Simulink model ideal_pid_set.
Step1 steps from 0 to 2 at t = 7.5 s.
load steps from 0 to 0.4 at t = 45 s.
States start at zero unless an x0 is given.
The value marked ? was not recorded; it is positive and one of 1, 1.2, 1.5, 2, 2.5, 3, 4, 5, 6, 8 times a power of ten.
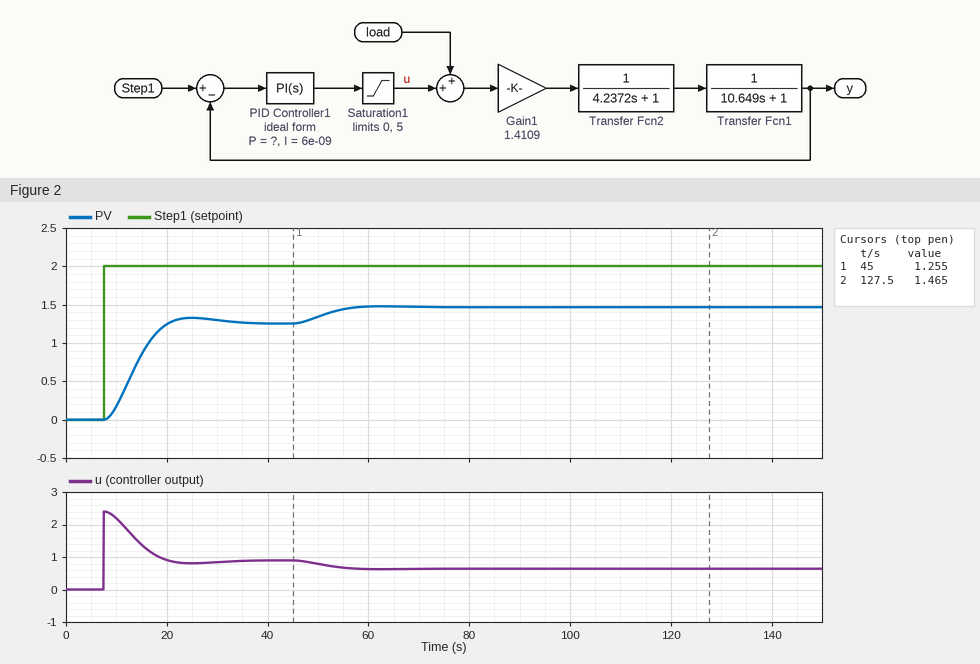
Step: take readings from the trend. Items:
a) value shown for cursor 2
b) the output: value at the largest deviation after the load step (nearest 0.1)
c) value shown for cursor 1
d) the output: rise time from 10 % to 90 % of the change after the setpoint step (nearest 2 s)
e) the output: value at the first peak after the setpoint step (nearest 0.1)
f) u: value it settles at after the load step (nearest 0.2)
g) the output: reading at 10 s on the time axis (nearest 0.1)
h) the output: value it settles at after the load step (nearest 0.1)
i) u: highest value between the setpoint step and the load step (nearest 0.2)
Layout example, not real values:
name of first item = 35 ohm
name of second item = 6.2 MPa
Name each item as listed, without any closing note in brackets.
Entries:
value shown for cursor 2 = 1.465
the output: value at the largest deviation after the load step = 1.5
value shown for cursor 1 = 1.255
the output: rise time from 10 % to 90 % of the change after the setpoint step = 8 s
the output: value at the first peak after the setpoint step = 1.3
u: value it settles at after the load step = 0.6
the output: reading at 10 s on the time axis = 0.2
the output: value it settles at after the load step = 1.5
u: highest value between the setpoint step and the load step = 2.4
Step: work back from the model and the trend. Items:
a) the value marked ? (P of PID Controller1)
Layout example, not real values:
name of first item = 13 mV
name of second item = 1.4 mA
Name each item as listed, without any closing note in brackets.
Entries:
the value marked ? = 1.2
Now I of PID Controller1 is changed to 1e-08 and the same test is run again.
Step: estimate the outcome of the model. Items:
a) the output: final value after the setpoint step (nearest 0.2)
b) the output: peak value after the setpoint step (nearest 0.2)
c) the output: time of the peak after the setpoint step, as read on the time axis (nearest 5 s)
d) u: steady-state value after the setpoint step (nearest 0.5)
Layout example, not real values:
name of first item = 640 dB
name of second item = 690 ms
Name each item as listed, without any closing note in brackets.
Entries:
the output: final value after the setpoint step = 1.2
the output: peak value after the setpoint step = 1.4
the output: time of the peak after the setpoint step, as read on the time axis = 25 s
u: steady-state value after the setpoint step = 1.0
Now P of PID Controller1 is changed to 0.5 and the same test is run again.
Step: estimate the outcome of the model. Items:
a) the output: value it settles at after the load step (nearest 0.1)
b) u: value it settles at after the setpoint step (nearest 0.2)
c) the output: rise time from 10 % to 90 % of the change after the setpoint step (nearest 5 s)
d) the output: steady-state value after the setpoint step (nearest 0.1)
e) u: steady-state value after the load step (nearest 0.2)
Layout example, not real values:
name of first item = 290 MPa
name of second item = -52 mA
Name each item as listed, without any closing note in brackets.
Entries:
the output: value it settles at after the load step = 1.2
u: value it settles at after the setpoint step = 0.6
the output: rise time from 10 % to 90 % of the change after the setpoint step = 15 s
the output: steady-state value after the setpoint step = 0.8
u: steady-state value after the load step = 0.4
